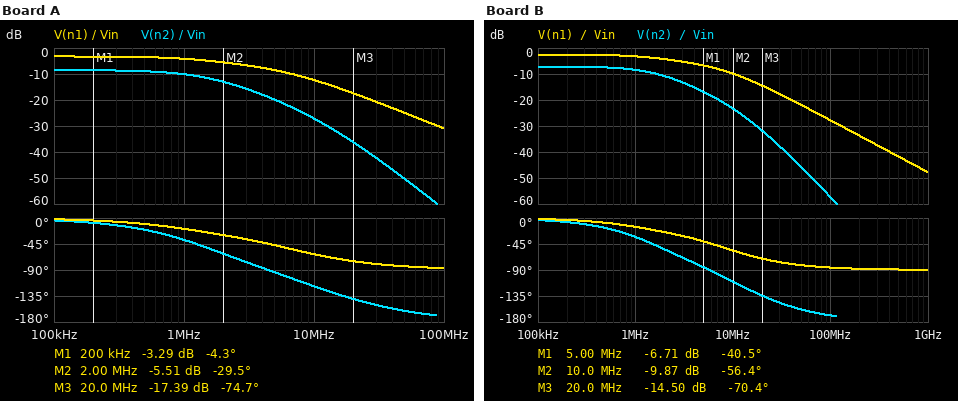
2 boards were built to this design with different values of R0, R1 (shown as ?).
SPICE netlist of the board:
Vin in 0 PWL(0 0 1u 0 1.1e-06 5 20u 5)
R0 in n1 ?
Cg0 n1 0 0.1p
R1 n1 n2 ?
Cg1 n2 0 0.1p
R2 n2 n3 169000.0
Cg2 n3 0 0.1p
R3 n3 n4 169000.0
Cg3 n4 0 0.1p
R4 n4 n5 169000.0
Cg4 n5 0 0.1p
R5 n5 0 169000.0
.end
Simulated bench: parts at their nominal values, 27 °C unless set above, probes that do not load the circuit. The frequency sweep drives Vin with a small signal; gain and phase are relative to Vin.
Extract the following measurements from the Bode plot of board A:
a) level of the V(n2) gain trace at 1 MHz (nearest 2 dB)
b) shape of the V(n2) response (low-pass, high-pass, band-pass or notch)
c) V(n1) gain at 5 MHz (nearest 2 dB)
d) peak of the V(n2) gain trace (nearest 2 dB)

-10 dB
low-pass
-8 dB
-8 dB
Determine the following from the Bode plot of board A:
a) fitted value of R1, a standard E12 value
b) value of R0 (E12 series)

560 kΩ
560 kΩ
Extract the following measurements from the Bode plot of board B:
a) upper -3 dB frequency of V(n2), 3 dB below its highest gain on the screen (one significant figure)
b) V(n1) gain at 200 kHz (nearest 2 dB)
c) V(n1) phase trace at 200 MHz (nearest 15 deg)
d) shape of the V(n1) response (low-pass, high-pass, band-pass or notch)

2 MHz
-2 dB
-90 deg
low-pass
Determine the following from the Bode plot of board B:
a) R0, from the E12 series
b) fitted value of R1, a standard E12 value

390 kΩ
470 kΩ
